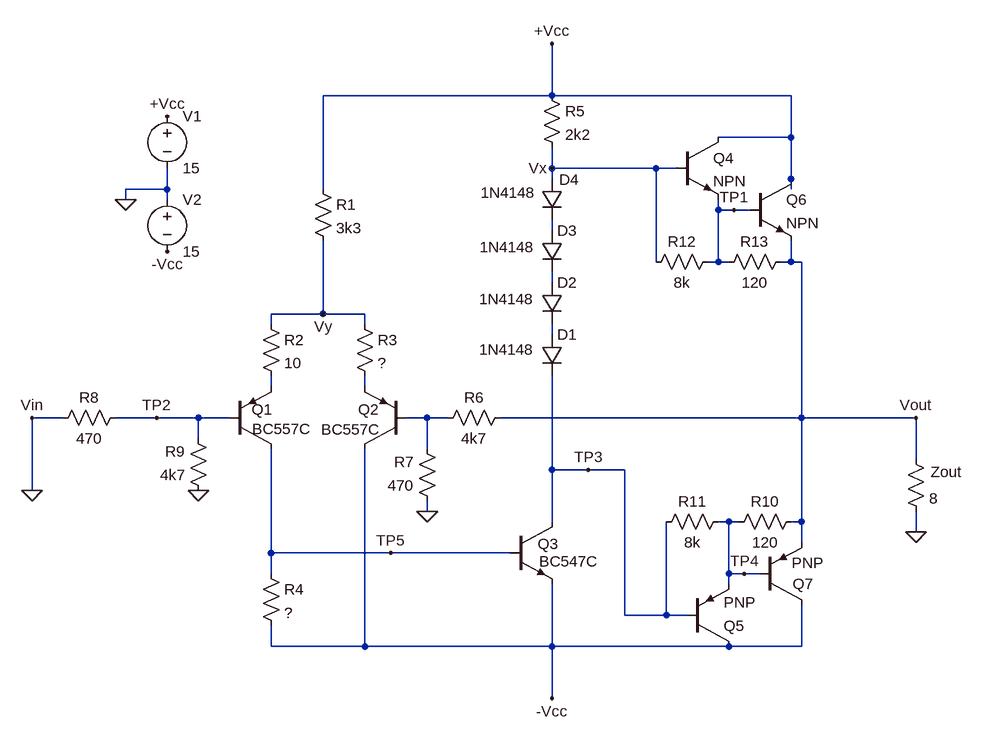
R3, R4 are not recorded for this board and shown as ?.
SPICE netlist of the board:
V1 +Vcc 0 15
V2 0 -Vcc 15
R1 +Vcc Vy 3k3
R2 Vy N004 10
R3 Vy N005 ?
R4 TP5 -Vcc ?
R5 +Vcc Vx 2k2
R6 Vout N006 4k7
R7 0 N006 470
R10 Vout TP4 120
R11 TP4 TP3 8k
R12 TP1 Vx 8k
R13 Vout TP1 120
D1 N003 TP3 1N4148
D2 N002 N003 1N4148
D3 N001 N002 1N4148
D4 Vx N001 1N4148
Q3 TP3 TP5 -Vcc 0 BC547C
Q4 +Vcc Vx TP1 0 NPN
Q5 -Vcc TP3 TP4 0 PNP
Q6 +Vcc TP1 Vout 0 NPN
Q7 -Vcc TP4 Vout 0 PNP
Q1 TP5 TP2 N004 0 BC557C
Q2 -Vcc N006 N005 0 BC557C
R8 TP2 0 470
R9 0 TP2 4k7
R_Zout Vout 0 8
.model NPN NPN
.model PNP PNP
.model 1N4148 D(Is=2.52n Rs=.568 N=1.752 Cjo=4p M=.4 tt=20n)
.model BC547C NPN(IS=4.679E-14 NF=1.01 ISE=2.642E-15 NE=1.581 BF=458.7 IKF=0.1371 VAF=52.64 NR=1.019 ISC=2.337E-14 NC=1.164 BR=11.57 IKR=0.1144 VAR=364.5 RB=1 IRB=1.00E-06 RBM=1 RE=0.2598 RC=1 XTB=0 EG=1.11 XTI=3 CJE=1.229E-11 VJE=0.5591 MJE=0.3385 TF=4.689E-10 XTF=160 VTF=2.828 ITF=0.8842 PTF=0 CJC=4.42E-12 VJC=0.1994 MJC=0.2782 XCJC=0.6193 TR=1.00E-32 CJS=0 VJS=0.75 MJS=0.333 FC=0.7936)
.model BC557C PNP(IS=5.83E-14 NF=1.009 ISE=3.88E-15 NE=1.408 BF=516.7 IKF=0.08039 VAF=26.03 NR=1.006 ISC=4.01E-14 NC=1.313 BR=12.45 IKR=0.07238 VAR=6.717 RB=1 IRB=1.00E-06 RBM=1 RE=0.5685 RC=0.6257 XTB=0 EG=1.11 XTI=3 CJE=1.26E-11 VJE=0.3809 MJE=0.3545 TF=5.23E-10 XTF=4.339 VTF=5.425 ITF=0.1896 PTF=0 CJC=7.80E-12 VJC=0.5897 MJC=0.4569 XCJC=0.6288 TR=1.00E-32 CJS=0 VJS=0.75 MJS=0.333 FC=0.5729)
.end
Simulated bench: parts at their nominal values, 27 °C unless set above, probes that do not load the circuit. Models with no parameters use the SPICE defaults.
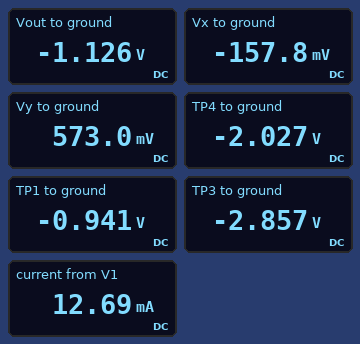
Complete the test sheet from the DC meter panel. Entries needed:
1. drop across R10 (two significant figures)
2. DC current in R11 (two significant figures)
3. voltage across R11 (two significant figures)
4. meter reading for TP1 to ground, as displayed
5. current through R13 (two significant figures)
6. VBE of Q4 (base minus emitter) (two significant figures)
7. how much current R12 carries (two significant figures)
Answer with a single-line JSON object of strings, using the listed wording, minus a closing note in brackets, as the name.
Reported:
{"drop across R10": "900 mV", "DC current in R11": "100 µA", "voltage across R11": "830 mV", "meter reading for TP1 to ground, as displayed": "-0.941 V", "current through R13": "1.5 mA", "VBE of Q4 (base minus emitter)": "780 mV", "how much current R12 carries": "98 µA"}
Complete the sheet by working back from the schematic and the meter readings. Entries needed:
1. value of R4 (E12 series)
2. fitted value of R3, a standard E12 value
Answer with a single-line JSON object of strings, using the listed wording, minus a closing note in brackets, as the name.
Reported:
{"value of R4": "2.7 kΩ", "fitted value of R3, a standard E12 value": "6.8 Ω"}
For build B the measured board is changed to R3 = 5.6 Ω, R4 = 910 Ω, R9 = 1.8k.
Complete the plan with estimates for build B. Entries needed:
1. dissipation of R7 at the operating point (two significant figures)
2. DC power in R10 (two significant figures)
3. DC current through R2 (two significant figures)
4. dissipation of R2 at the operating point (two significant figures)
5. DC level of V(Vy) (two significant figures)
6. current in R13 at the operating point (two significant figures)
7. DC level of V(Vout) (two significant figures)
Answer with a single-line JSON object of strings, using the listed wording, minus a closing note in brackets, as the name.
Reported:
{"dissipation of R7 at the operating point": "6.5 µW", "DC power in R10": "6.5 mW", "DC current through R2": "750 µA", "dissipation of R2 at the operating point": "5.6 µW", "DC level of V(Vy)": "610 mV", "current in R13 at the operating point": "1.6 mA", "DC level of V(Vout)": "-630 mV"}
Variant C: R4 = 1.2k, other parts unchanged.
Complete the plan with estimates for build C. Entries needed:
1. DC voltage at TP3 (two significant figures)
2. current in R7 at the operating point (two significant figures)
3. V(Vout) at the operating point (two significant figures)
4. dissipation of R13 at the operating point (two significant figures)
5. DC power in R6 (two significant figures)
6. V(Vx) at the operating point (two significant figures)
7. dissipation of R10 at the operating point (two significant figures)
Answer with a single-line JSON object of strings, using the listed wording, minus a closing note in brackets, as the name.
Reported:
{"DC voltage at TP3": "-2.5 V", "current in R7 at the operating point": "150 µA", "V(Vout) at the operating point": "-810 mV", "dissipation of R13 at the operating point": "300 µW", "DC power in R6": "120 µW", "V(Vx) at the operating point": "160 mV", "dissipation of R10 at the operating point": "6.6 mW"}
